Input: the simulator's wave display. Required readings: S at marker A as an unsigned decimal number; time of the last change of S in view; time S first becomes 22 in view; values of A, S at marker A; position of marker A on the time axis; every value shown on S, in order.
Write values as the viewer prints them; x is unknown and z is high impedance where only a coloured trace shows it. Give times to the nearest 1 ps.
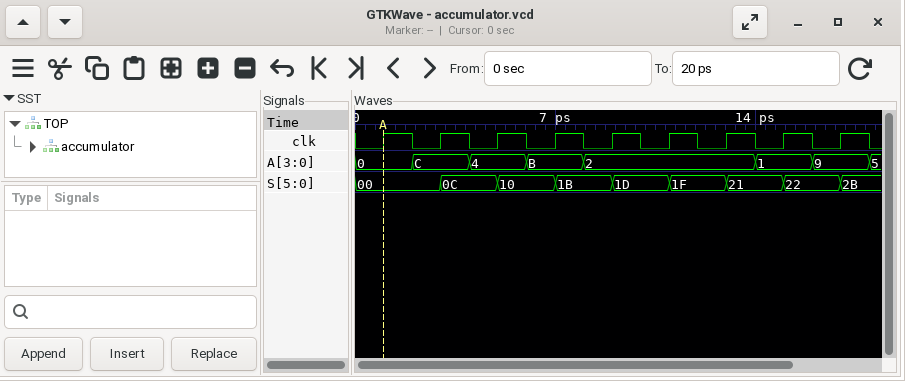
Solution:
0
17 ps
15 ps
A=0, S=00
1 ps
00, 0C, 10, 1B, 1D, 1F, 21, 22, 2B
